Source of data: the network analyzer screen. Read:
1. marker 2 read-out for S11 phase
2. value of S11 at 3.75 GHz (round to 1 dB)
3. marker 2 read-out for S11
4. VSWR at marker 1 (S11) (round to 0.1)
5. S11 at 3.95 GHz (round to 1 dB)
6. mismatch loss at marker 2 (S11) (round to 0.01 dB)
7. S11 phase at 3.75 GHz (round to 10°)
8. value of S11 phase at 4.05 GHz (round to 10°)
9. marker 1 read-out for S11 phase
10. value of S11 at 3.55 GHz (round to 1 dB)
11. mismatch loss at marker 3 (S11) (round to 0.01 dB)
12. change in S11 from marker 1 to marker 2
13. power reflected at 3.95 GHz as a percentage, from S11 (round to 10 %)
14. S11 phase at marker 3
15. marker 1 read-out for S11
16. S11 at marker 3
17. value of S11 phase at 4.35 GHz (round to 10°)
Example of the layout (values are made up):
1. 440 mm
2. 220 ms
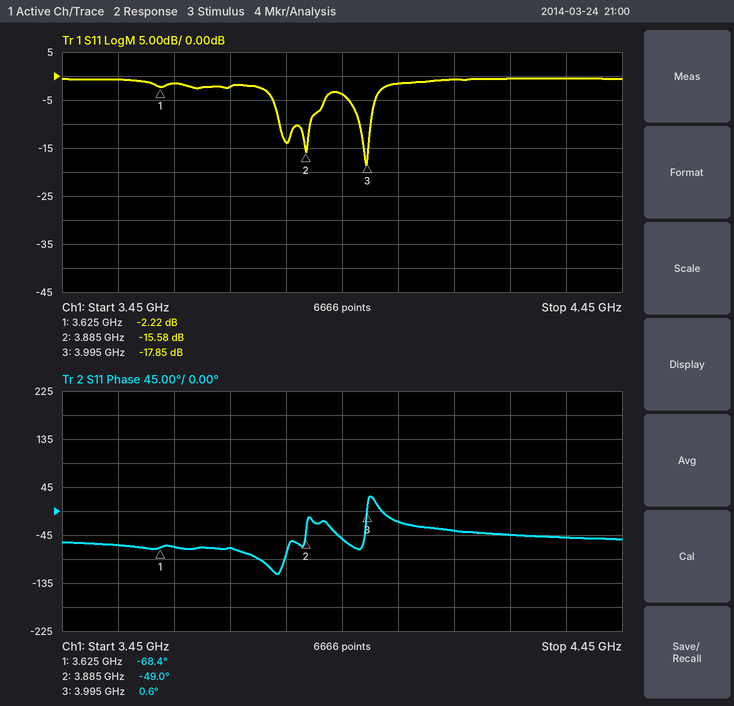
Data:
1. -49.0°
2. -2 dB
3. -15.58 dB
4. 7.9
5. -4 dB
6. 0.12 dB
7. -70°
8. -20°
9. -68.4°
10. -1 dB
11. 0.07 dB
12. -13.36 dB
13. 40 %
14. 0.6°
15. -2.22 dB
16. -17.85 dB
17. -50°
